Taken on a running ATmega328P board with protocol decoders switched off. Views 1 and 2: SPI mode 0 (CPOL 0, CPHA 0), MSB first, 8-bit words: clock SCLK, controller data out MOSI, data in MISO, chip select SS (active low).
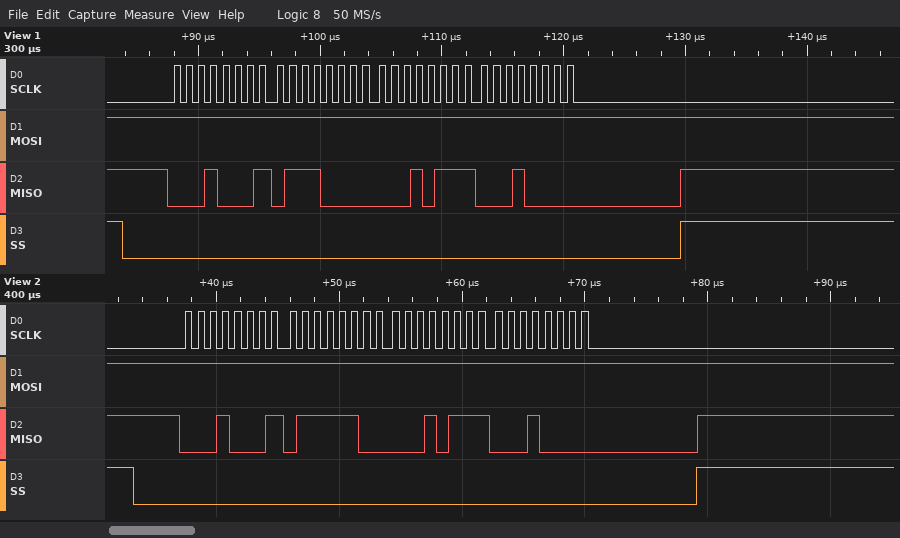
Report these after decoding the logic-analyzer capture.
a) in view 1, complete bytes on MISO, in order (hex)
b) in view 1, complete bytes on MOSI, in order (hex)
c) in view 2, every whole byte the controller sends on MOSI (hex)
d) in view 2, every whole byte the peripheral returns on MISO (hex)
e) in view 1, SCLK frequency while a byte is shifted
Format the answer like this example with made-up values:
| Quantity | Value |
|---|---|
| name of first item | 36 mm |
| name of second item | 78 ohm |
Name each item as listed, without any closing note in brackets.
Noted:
| Quantity | Value |
|---|---|
| in view 1, complete bytes on MISO, in order | 0x11 0x70 0x17 0x10 |
| in view 1, complete bytes on MOSI, in order | 0xFF 0xFF 0xFF 0xFF |
| in view 2, every whole byte the controller sends on MOSI | 0xFF 0xFF 0xFF 0xFF |
| in view 2, every whole byte the peripheral returns on MISO | 0x11 0x7C 0x17 0x10 |
| in view 1, SCLK frequency while a byte is shifted | 1 MHz |
